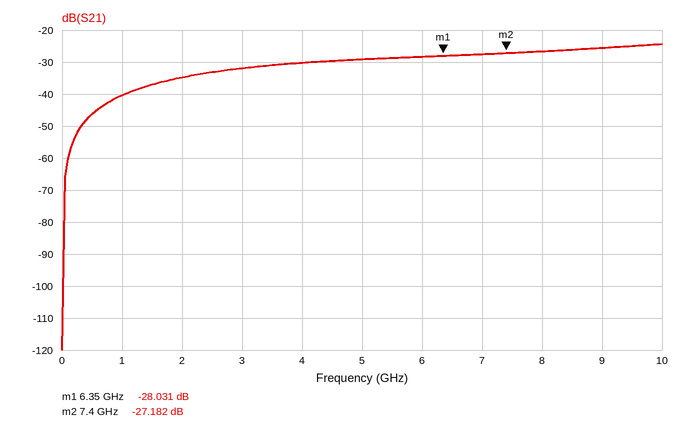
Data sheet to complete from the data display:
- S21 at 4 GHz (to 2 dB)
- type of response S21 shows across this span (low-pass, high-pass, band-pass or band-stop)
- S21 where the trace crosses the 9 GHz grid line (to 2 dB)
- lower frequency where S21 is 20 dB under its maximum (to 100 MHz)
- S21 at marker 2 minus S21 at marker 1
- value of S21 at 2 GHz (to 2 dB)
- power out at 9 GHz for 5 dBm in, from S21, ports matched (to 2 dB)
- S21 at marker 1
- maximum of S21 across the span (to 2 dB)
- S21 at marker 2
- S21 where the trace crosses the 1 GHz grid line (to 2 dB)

-30 dB
high-pass
-26 dB
600 MHz
0.849 dB
-34 dB
-20 dBm
-28.031 dB
-24 dB
-27.182 dB
-40 dB
